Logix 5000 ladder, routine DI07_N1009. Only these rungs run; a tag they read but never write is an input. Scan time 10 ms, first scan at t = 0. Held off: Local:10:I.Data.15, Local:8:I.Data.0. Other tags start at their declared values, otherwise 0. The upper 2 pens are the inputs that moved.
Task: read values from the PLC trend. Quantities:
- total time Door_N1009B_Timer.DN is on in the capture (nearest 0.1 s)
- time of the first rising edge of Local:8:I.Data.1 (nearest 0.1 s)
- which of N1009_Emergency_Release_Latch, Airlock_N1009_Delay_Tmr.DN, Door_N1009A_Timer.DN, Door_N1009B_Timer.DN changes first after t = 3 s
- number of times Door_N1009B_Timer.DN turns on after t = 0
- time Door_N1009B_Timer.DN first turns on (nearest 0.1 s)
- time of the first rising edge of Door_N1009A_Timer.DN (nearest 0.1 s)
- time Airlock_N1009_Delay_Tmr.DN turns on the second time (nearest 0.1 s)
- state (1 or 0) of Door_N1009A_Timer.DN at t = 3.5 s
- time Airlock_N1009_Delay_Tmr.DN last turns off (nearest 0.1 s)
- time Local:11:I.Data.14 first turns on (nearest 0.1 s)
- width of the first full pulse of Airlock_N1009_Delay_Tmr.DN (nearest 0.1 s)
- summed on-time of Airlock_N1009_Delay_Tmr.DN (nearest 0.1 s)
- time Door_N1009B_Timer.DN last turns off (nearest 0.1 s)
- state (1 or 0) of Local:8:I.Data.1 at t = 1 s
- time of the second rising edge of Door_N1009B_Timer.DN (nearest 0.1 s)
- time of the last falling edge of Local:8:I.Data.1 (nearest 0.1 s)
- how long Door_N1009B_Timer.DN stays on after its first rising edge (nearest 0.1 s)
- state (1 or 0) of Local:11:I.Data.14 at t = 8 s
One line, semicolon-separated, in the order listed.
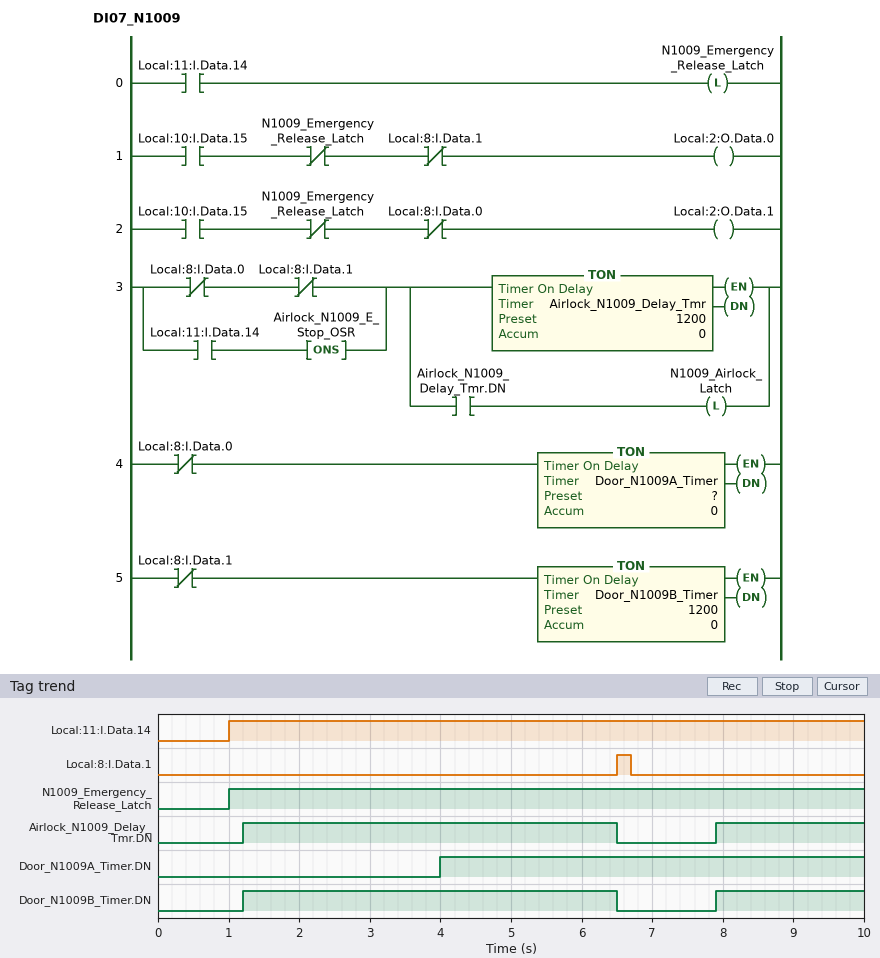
7.4 s; 6.5 s; Door_N1009A_Timer.DN; 2; 1.2 s; 4.0 s; 7.9 s; 0; 6.5 s; 1.0 s; 5.3 s; 7.4 s; 6.5 s; 0; 7.9 s; 6.7 s; 5.3 s; 1
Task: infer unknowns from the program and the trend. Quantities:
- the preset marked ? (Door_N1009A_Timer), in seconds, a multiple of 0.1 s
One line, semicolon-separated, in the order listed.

4.0 s
